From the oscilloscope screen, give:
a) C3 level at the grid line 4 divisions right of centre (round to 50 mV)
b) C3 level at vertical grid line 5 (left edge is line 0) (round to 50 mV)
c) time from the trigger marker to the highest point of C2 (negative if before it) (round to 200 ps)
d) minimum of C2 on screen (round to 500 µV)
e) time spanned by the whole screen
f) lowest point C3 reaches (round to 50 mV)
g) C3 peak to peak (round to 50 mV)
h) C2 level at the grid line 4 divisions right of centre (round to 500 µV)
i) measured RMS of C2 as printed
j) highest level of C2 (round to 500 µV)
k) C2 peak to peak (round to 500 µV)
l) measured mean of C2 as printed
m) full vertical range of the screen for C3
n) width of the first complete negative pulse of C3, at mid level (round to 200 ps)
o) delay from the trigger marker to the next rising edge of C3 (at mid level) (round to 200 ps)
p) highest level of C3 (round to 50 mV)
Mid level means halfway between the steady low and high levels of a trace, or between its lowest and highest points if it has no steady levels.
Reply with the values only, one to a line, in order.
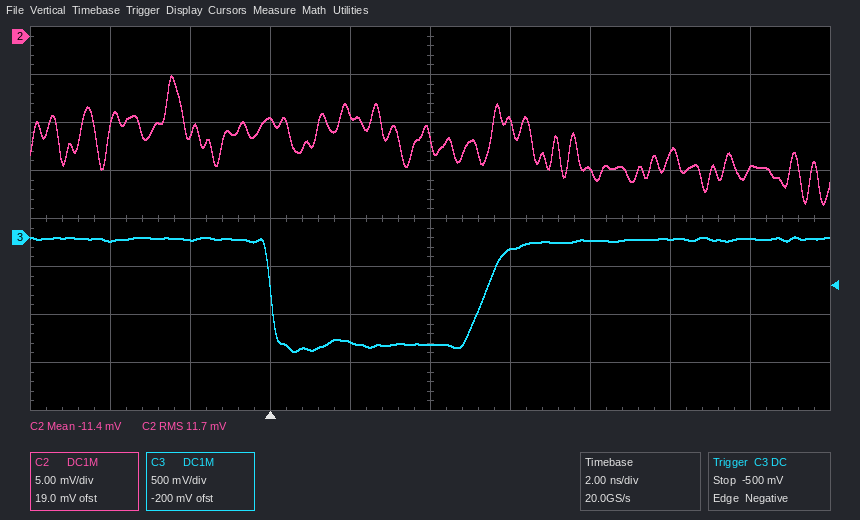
0 mV
-1.10 V
-2.4 ns
-17.5 mV
20 ns
-1.20 V
1.20 V
-14.0 mV
11.7 mV
-4.0 mV
13.5 mV
-11.4 mV
4 V
5.4 ns
5.4 ns
0 mV
